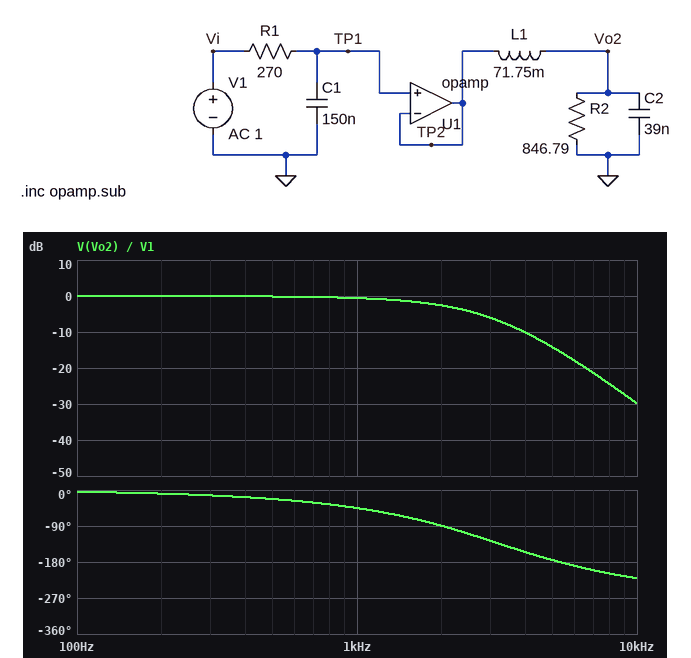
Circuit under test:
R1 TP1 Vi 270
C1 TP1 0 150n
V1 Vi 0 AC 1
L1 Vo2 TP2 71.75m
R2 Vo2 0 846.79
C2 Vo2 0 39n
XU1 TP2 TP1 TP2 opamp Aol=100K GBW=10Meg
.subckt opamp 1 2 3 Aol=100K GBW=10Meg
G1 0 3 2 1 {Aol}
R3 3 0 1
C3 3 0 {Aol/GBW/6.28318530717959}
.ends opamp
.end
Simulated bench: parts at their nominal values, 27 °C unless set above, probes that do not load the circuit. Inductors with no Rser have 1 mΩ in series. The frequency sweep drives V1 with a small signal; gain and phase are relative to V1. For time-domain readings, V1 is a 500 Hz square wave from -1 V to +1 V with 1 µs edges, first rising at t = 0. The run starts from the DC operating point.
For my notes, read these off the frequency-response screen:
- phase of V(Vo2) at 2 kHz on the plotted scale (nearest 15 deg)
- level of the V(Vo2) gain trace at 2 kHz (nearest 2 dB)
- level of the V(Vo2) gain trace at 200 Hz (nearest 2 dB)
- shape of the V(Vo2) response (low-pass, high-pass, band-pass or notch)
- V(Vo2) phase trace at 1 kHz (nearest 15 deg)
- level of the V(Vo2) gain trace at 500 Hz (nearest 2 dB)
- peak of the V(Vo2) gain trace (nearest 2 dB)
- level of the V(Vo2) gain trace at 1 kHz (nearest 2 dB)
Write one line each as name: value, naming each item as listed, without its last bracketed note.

phase of V(Vo2) at 2 kHz on the plotted scale: -90 deg
level of the V(Vo2) gain trace at 2 kHz: -2 dB
level of the V(Vo2) gain trace at 200 Hz: 0 dB
shape of the V(Vo2) response: low-pass
V(Vo2) phase trace at 1 kHz: -45 deg
level of the V(Vo2) gain trace at 500 Hz: 0 dB
peak of the V(Vo2) gain trace: 0 dB
level of the V(Vo2) gain trace at 1 kHz: 0 dB
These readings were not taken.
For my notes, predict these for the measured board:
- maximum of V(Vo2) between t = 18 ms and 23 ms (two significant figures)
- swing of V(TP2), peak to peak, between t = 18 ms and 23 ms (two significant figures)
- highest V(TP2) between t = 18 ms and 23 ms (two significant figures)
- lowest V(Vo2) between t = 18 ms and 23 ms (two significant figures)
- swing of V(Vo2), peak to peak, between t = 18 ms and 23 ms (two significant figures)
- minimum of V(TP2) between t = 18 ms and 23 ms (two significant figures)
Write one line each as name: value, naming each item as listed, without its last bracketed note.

maximum of V(Vo2) between t = 18 ms and 23 ms: 1.0 V
swing of V(TP2), peak to peak, between t = 18 ms and 23 ms: 2.0 V
highest V(TP2) between t = 18 ms and 23 ms: 1.0 V
lowest V(Vo2) between t = 18 ms and 23 ms: -1.0 V
swing of V(Vo2), peak to peak, between t = 18 ms and 23 ms: 2.0 V
minimum of V(TP2) between t = 18 ms and 23 ms: -1.0 V
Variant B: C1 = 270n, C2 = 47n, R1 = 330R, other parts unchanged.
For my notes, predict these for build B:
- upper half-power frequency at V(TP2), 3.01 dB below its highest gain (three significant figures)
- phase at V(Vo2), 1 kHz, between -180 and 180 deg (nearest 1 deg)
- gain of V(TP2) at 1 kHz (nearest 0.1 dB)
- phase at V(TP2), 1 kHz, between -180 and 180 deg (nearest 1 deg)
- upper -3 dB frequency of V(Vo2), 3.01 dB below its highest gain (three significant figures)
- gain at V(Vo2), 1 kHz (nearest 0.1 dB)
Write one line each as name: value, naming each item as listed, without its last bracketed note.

upper half-power frequency at V(TP2), 3.01 dB below its highest gain: 1.79 kHz
phase at V(Vo2), 1 kHz, between -180 and 180 deg: -61 deg
gain of V(TP2) at 1 kHz: -1.2 dB
phase at V(TP2), 1 kHz, between -180 and 180 deg: -29 deg
upper -3 dB frequency of V(Vo2), 3.01 dB below its highest gain: 1.55 kHz
gain at V(Vo2), 1 kHz: -1.3 dB
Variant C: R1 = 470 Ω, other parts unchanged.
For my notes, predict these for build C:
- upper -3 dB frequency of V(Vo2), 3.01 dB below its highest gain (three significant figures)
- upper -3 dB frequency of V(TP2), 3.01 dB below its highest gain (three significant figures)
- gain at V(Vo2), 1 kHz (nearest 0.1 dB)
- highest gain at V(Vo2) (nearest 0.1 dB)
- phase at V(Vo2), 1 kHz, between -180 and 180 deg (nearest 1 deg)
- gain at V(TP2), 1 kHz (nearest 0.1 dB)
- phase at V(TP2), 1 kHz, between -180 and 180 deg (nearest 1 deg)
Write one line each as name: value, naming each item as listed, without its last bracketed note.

upper -3 dB frequency of V(Vo2), 3.01 dB below its highest gain: 1.69 kHz
upper -3 dB frequency of V(TP2), 3.01 dB below its highest gain: 2.26 kHz
gain at V(Vo2), 1 kHz: -1.1 dB
highest gain at V(Vo2): 0 dB
phase at V(Vo2), 1 kHz, between -180 and 180 deg: -55 deg
gain at V(TP2), 1 kHz: -0.8 dB
phase at V(TP2), 1 kHz, between -180 and 180 deg: -24 deg
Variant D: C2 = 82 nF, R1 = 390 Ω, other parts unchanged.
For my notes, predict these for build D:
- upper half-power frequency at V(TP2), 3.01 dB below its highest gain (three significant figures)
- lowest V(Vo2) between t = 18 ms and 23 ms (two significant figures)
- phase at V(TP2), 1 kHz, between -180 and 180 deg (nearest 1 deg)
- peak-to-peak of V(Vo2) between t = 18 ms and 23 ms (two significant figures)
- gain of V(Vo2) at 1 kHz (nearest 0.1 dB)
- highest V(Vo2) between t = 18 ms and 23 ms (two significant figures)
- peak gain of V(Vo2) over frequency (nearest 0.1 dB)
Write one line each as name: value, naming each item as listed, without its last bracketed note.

upper half-power frequency at V(TP2), 3.01 dB below its highest gain: 2.72 kHz
lowest V(Vo2) between t = 18 ms and 23 ms: -1.2 V
phase at V(TP2), 1 kHz, between -180 and 180 deg: -20 deg
peak-to-peak of V(Vo2) between t = 18 ms and 23 ms: 2.3 V
gain of V(Vo2) at 1 kHz: 0 dB
highest V(Vo2) between t = 18 ms and 23 ms: 1.2 V
peak gain of V(Vo2) over frequency: 0.1 dB
